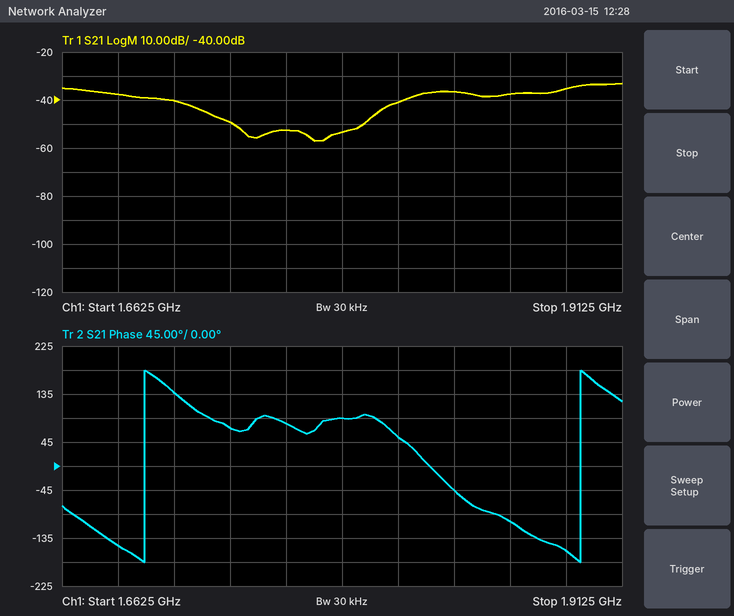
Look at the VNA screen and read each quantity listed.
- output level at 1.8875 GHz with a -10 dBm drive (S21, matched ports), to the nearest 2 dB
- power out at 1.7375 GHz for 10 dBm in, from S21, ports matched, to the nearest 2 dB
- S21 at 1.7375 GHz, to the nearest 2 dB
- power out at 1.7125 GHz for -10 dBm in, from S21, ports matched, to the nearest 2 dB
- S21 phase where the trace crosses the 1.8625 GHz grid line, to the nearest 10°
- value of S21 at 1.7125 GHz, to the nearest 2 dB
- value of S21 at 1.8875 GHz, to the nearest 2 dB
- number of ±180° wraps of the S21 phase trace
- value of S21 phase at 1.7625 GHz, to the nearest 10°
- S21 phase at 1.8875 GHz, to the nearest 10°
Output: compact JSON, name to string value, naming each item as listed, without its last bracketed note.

{"output level at 1.8875 GHz with a -10 dBm drive (S21, matched ports), to the nearest 2 dB": "-46 dBm", "power out at 1.7375 GHz for 10 dBm in, from S21, ports matched, to the nearest 2 dB": "-40 dBm", "S21 at 1.7375 GHz, to the nearest 2 dB": "-50 dB", "power out at 1.7125 GHz for -10 dBm in, from S21, ports matched, to the nearest 2 dB": "-50 dBm", "S21 phase where the trace crosses the 1.8625 GHz grid line, to the nearest 10°": "-100°", "value of S21 at 1.7125 GHz, to the nearest 2 dB": "-40 dB", "value of S21 at 1.8875 GHz, to the nearest 2 dB": "-36 dB", "number of ±180° wraps of the S21 phase trace": "2", "value of S21 phase at 1.7625 GHz, to the nearest 10°": "80°", "S21 phase at 1.8875 GHz, to the nearest 10°": "-160°"}
